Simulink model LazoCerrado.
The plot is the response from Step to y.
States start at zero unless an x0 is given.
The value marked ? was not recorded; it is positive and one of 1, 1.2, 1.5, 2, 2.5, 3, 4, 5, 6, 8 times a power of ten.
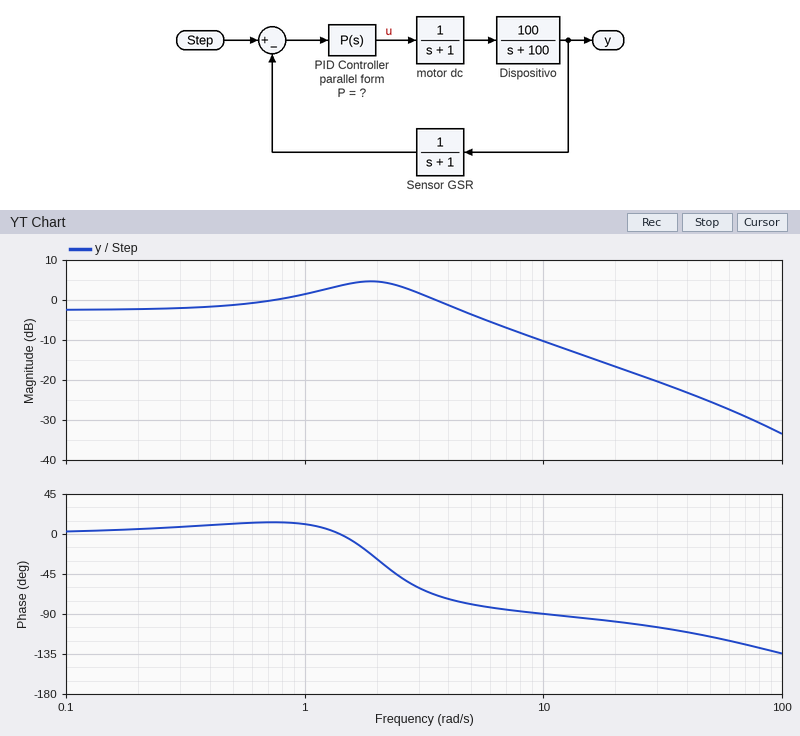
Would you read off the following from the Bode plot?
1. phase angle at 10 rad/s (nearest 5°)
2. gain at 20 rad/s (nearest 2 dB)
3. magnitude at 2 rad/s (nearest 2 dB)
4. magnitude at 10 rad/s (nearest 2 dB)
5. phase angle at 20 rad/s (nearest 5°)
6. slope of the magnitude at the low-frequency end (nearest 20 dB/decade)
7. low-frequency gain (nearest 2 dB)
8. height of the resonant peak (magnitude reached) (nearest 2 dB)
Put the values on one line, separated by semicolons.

-90°; -16 dB; 4 dB; -10 dB; -100°; 0 dB/decade; -2 dB; 4 dB
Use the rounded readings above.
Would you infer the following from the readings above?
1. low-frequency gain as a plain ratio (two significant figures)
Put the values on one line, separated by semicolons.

0.79
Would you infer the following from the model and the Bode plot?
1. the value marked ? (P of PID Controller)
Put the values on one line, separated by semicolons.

3
